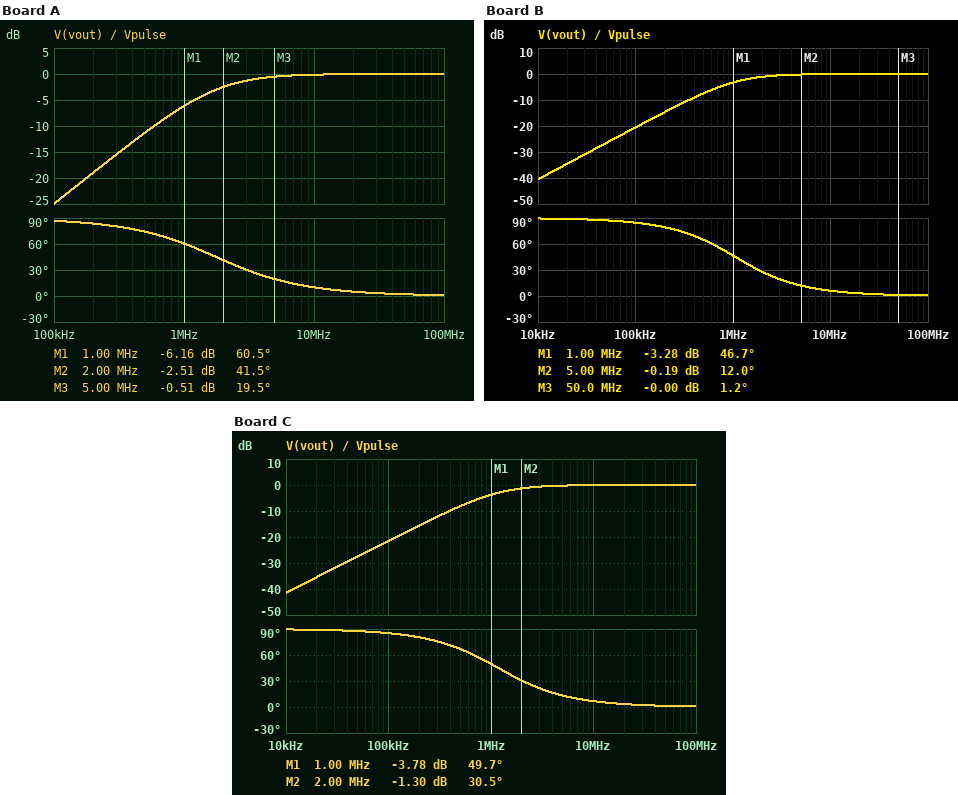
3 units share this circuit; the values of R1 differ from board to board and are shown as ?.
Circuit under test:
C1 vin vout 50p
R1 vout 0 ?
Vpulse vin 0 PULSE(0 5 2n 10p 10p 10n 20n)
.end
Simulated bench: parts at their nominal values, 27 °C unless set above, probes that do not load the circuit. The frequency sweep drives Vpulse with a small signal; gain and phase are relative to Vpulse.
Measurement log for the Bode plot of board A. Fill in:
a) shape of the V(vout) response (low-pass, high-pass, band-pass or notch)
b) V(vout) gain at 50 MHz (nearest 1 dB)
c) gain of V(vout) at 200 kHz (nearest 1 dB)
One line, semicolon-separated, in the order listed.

high-pass; 0 dB; -19 dB
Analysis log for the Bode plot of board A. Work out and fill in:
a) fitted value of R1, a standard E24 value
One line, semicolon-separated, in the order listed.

1.8 kΩ
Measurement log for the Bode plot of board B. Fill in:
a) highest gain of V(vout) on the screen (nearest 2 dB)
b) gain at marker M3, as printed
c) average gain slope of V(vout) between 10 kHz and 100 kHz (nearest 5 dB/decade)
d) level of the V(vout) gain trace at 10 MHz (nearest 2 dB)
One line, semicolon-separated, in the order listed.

0 dB; -0.00 dB; 20 dB/decade; 0 dB
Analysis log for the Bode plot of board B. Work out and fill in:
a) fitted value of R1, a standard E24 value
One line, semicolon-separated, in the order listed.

3 kΩ
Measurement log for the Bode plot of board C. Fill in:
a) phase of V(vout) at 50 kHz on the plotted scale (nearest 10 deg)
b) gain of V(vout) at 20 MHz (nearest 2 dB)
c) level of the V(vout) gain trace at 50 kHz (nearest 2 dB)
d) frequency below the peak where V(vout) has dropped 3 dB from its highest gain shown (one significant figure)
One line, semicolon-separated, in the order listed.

90 deg; 0 dB; -28 dB; 1 MHz
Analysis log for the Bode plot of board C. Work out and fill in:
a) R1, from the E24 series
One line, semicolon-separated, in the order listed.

2.7 kΩ
